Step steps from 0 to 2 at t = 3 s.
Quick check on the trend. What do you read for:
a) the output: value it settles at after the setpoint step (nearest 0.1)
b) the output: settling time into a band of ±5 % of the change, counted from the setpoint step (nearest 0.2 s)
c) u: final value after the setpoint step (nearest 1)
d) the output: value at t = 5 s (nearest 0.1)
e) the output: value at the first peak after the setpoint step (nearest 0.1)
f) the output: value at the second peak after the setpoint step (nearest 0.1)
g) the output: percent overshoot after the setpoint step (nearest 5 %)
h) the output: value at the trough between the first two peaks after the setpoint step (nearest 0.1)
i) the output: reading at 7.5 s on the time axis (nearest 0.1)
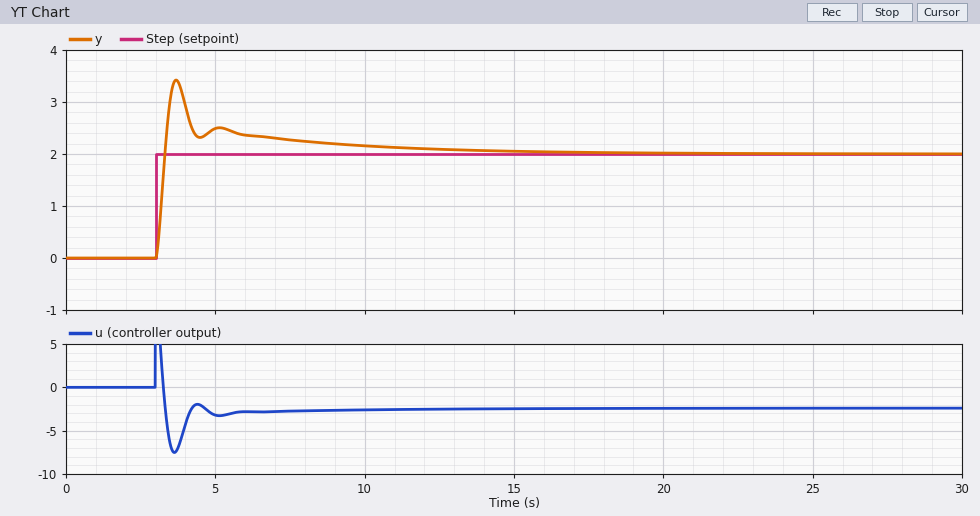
2.0
9.0 s
-2
2.5
3.4
2.5
70 %
2.3
2.3
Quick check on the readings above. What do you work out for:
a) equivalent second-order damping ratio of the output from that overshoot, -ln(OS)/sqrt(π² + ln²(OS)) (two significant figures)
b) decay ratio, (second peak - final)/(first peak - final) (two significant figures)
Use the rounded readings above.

0.11
0.36
